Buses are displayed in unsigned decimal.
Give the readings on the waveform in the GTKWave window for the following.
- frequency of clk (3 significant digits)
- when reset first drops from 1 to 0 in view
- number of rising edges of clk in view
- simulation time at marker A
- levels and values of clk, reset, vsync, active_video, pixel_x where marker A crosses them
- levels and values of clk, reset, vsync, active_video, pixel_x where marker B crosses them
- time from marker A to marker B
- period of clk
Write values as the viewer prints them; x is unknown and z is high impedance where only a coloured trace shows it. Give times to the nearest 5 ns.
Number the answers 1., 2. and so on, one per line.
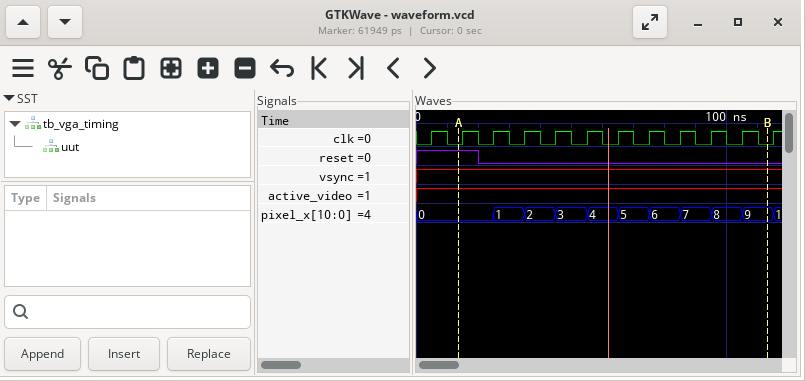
1. 100 MHz
2. 20 ns
3. 12
4. 15 ns
5. clk=0, reset=1, vsync=1, active_video=1, pixel_x=0
6. clk=0, reset=0, vsync=1, active_video=1, pixel_x=9
7. 100 ns
8. 10 ns
